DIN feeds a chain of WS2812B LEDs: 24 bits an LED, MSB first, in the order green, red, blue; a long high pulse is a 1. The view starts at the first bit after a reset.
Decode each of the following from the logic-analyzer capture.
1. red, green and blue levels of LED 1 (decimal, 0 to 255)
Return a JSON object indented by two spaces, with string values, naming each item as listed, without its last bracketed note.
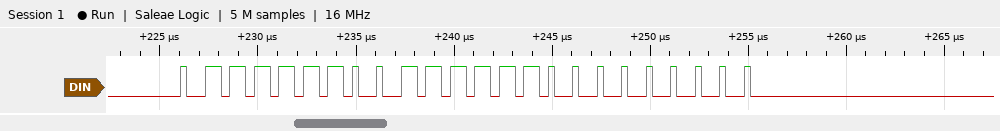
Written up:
{
  "red, green and blue levels of LED 1": "126, 126, 0"
}
